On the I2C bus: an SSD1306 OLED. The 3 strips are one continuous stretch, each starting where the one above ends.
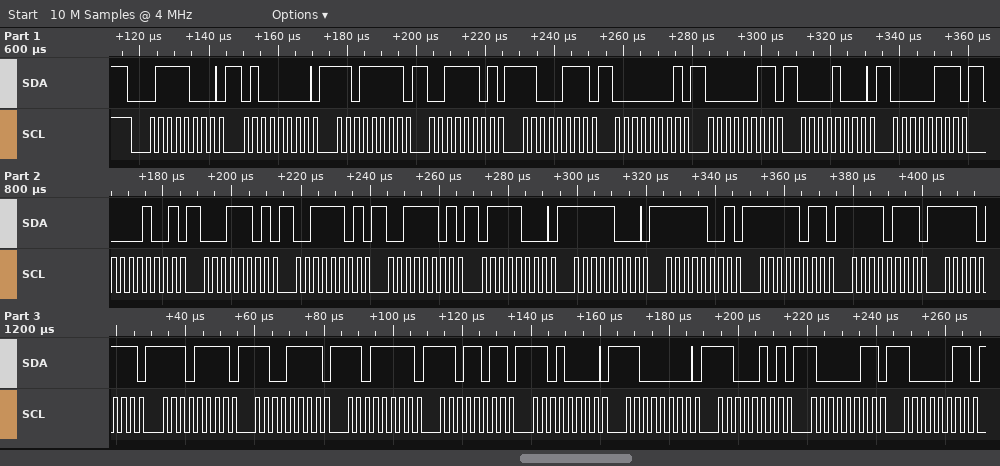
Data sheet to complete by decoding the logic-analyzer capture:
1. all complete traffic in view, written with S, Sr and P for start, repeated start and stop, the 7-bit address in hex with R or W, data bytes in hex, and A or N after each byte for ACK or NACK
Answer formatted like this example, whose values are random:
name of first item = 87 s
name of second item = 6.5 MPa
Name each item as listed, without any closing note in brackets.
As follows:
all complete traffic in view, written with S, Sr and P for start, repeated start and stop, the 7-bit address in hex with R or W, data bytes in hex, and A or N after each byte for ACK or NACK = S 3CW A 40 A DF A 3D A C7 A 01 A 03 A 08 A 07 A 09 A 1D A 3D A 3D A 78 A F8 A F9 A FB A F7 A F7 A EF A CF A DF A DB A D0 A C0 A C5 A 83 A 83 A
